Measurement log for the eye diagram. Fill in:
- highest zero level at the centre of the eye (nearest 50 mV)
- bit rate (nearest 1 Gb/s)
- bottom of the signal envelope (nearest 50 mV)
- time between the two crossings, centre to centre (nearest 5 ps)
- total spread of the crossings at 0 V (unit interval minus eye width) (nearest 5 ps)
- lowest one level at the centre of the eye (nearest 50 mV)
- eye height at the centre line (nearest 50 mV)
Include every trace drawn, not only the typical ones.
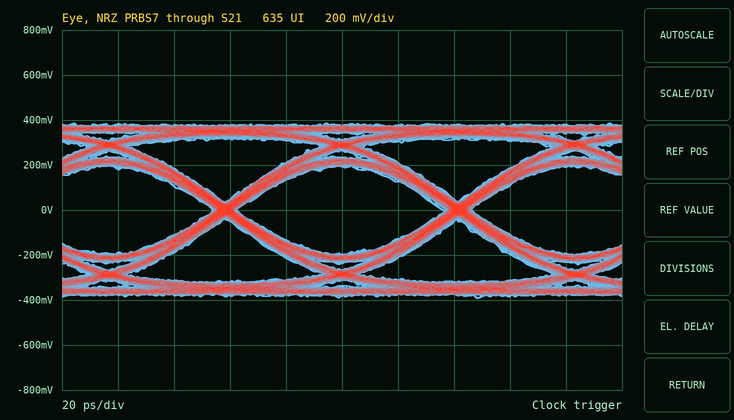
-200 mV
12 Gb/s
-400 mV
85 ps
10 ps
200 mV
400 mV
